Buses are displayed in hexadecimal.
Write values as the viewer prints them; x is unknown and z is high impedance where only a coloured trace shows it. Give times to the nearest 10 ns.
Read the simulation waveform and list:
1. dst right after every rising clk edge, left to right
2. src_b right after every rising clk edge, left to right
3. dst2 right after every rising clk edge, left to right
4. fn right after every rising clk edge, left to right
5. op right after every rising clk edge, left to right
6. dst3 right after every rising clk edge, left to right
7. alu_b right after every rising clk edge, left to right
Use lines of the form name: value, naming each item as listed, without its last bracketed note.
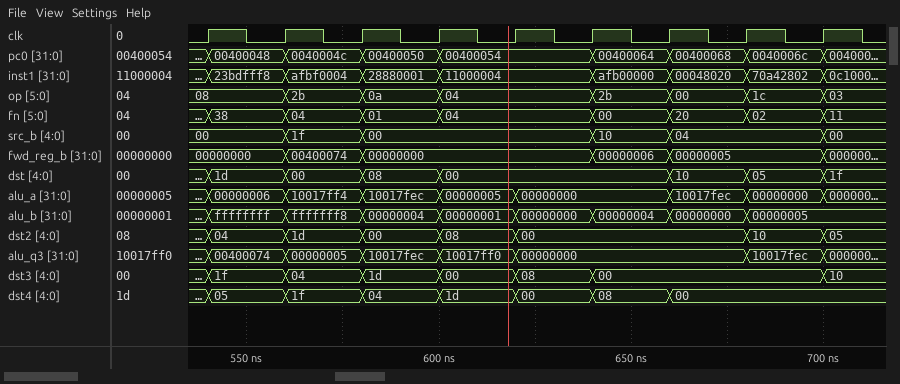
dst right after every rising clk edge, left to right: 1d, 00, 08, 00, 00, 00, 10, 05, 1f
src_b right after every rising clk edge, left to right: 00, 1f, 00, 00, 00, 10, 04, 04, 00
dst2 right after every rising clk edge, left to right: 04, 1d, 00, 08, 00, 00, 00, 10, 05
fn right after every rising clk edge, left to right: 38, 04, 01, 04, 04, 00, 20, 02, 11
op right after every rising clk edge, left to right: 08, 2b, 0a, 04, 04, 2b, 00, 1c, 03
dst3 right after every rising clk edge, left to right: 1f, 04, 1d, 00, 08, 00, 00, 00, 10
alu_b right after every rising clk edge, left to right: ffffffff, fffffff8, 00000004, 00000001, 00000000, 00000004, 00000000, 00000005, 00000005
